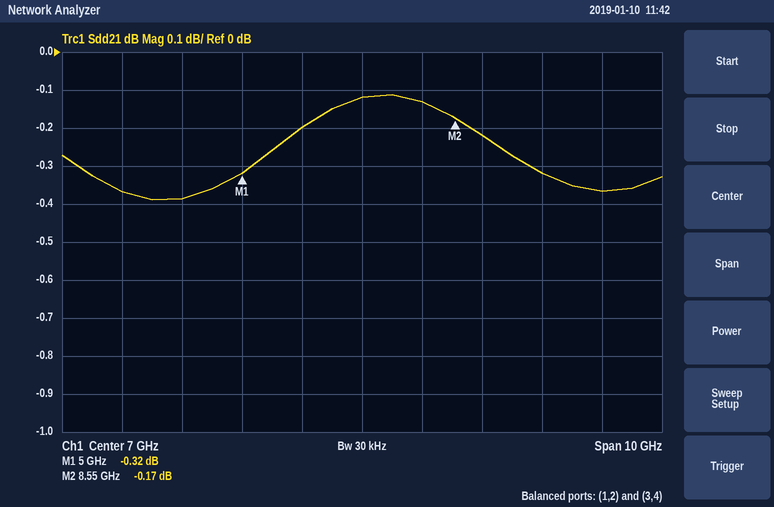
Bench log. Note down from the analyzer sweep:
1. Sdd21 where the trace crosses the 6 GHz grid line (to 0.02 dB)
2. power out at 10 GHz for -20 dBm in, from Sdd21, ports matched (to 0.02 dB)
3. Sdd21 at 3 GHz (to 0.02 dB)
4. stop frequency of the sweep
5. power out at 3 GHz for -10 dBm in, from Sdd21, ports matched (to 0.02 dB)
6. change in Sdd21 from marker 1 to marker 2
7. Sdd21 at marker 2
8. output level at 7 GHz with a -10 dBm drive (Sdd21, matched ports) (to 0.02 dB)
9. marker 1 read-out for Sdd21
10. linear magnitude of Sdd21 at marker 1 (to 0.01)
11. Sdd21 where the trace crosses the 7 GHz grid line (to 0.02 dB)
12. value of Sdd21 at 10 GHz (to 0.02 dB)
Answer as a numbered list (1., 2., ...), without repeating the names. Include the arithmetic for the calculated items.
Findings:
1. -0.20 dB
2. -20 dBm + (-0.32 dB) = -20.32 dBm
3. -0.36 dB
4. 12 GHz
5. -10 dBm + (-0.36 dB) = -10.36 dBm
6. -0.17 − (-0.32) = 0.15 dB
7. -0.17 dB
8. -10 dBm + (-0.12 dB) = -10.12 dBm
9. -0.32 dB
10. 10^(-0.32/20) ≈ 0.96
11. -0.12 dB
12. -0.32 dB
